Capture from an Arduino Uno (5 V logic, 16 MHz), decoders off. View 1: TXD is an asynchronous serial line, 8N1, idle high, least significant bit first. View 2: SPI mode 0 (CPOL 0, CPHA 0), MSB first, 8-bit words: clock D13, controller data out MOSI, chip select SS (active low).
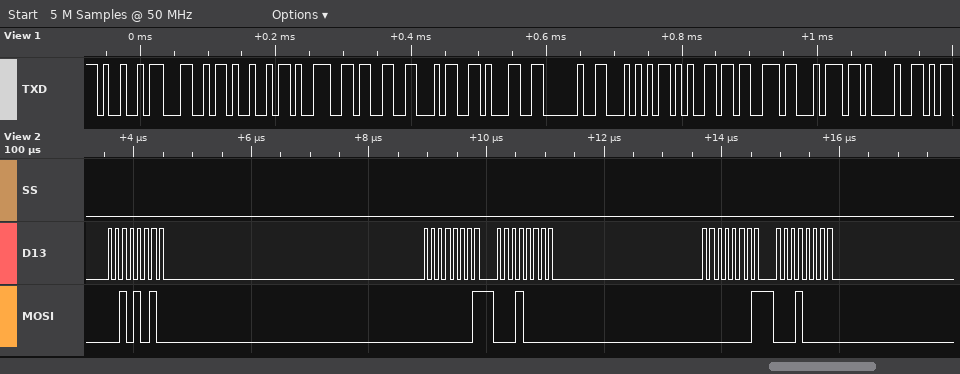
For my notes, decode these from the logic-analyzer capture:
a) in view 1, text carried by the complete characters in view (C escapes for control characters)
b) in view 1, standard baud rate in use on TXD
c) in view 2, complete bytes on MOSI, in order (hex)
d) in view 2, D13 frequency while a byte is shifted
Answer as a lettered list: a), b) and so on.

a) "ILI9341 Test!"
b) 115200 baud
c) 2A 01 10 01 10
d) 8 MHz
